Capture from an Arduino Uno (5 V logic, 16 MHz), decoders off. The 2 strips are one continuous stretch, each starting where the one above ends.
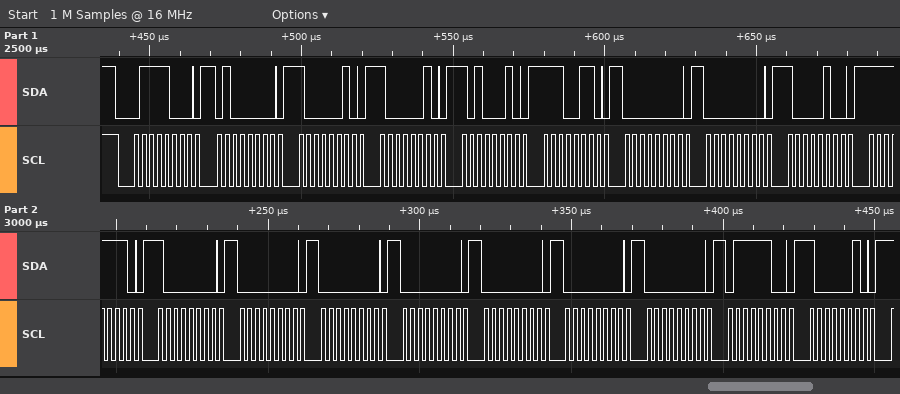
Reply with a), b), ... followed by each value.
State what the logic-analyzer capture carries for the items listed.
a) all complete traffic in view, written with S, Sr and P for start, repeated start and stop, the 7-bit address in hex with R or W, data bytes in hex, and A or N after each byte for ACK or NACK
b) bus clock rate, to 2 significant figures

a) S 3CW A 40 A 82 A 82 A A2 A E6 A 00 A 00 A 84 A FE A 80 A 00 A 00 A 00 A 00 A 00 A 00 A 7C A 82 A
b) 400 kHz
